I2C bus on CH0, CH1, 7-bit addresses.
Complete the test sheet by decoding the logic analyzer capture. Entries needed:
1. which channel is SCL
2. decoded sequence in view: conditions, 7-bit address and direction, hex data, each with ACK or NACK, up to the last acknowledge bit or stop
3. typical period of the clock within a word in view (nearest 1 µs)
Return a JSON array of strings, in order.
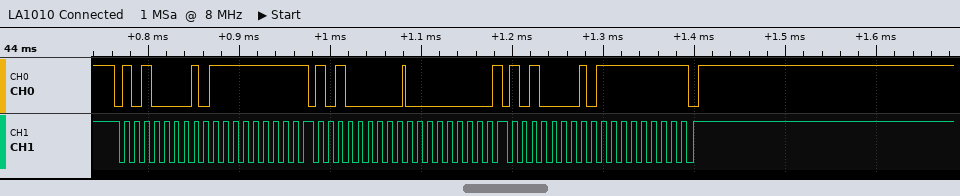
["CH1", "start, address 50 read ACK, FF NACK, repeated start, address 50 write ACK, 00 ACK, repeated start, address 50 read ACK, FF NACK, stop", "11 µs"]
